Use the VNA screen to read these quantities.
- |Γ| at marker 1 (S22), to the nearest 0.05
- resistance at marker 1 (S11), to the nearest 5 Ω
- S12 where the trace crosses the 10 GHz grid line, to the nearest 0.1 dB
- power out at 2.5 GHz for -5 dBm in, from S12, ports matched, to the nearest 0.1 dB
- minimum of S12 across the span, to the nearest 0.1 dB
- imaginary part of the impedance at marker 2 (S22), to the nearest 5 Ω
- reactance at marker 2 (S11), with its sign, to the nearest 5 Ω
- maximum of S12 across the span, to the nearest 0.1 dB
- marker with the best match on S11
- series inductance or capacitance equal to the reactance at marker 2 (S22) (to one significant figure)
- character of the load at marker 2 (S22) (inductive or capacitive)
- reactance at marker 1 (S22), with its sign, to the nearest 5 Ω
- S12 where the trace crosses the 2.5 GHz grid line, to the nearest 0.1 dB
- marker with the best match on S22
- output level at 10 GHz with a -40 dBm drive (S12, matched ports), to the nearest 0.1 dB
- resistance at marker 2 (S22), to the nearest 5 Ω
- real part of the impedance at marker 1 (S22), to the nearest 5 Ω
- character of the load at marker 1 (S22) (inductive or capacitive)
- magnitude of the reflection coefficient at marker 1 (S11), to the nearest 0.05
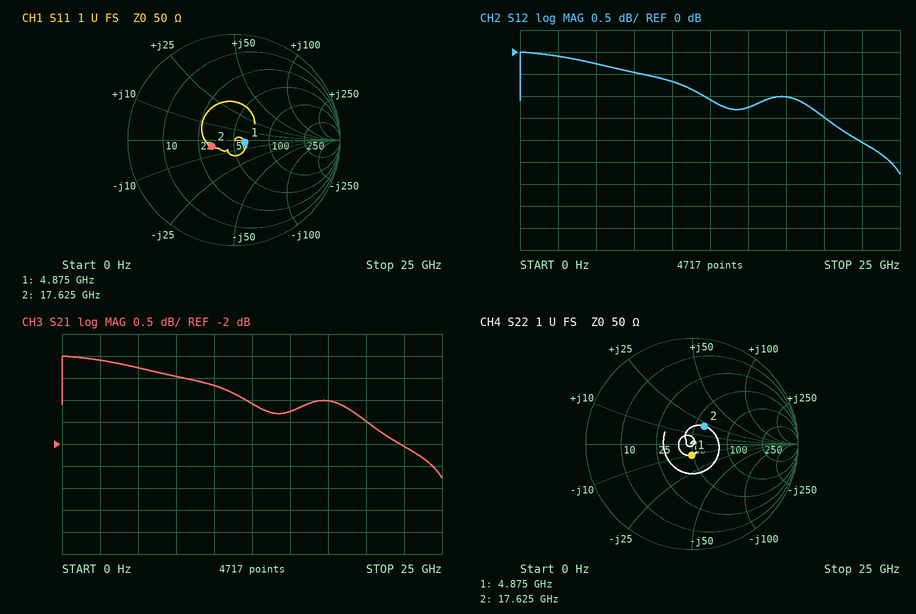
0.10
60 Ω
-0.7 dB
-5.1 dBm
-2.8 dB
+20 Ω
-5 Ω
0.0 dB
marker 1
200 pH
inductive
-10 Ω
-0.1 dB
marker 1
-40.7 dBm
60 Ω
50 Ω
capacitive
0.10
